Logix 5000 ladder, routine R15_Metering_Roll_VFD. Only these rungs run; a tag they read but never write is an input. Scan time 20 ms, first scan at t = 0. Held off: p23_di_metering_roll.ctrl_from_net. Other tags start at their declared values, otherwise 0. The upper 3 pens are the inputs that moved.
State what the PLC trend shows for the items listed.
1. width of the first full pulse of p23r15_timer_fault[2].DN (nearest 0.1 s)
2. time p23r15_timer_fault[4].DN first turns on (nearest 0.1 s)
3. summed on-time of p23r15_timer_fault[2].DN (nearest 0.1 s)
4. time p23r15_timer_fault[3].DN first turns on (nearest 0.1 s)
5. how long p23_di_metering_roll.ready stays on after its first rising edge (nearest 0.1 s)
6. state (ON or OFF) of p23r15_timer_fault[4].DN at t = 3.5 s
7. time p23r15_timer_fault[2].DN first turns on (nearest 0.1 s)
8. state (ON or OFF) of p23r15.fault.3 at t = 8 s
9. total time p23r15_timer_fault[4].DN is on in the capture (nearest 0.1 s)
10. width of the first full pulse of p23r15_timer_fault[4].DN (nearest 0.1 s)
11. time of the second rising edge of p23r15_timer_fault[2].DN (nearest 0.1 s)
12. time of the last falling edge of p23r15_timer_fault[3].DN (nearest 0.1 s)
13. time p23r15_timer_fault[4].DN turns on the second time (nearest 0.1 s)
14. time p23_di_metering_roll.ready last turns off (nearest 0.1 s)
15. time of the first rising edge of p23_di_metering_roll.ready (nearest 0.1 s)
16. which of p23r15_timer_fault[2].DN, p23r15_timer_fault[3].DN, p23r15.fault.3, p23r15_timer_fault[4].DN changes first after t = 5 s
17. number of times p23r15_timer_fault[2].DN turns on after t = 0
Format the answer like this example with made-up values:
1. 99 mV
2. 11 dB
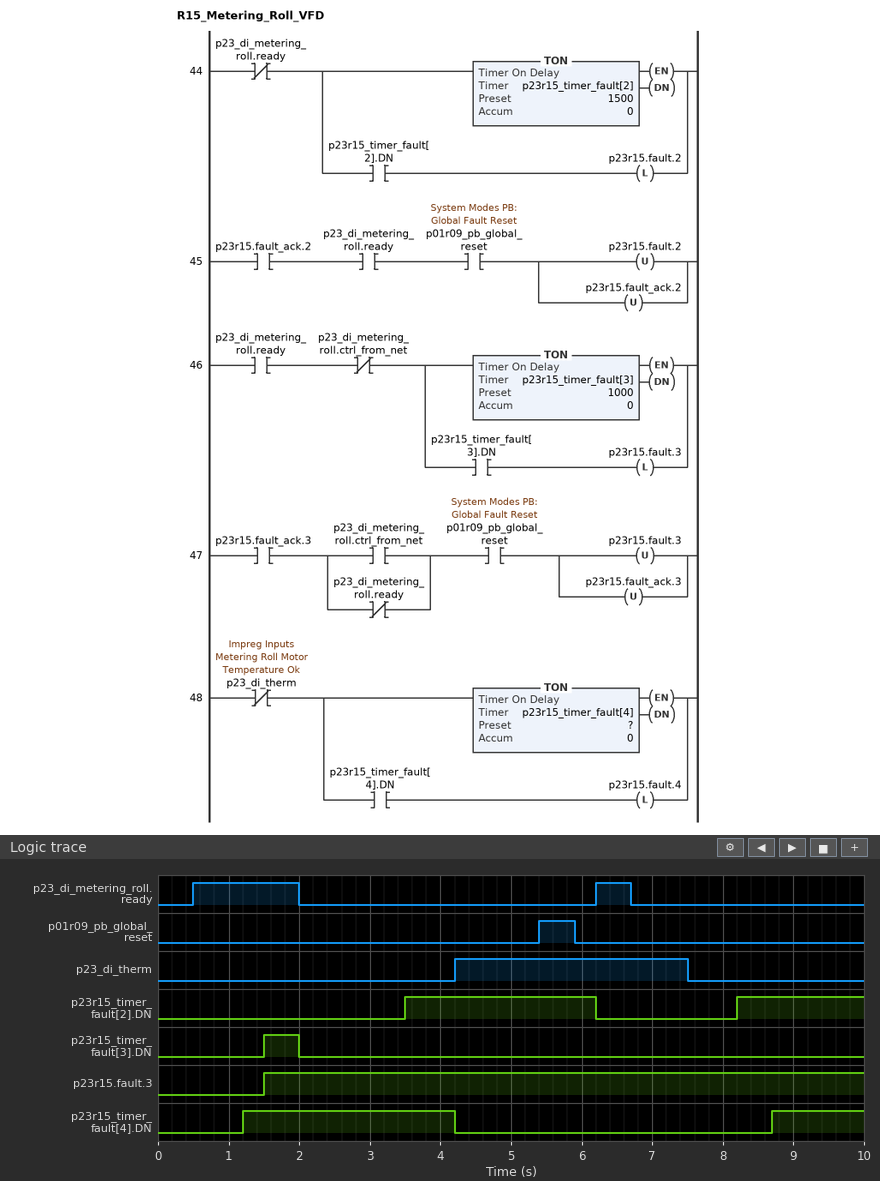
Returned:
1. 2.7 s
2. 1.2 s
3. 4.5 s
4. 1.5 s
5. 1.5 s
6. ON
7. 3.5 s
8. ON
9. 4.3 s
10. 3.0 s
11. 8.2 s
12. 2.0 s
13. 8.7 s
14. 6.7 s
15. 0.5 s
16. p23r15_timer_fault[2].DN
17. 2
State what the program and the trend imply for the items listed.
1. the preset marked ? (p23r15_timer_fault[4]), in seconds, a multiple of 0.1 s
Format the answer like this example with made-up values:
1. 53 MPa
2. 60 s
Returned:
1. 1.2 s
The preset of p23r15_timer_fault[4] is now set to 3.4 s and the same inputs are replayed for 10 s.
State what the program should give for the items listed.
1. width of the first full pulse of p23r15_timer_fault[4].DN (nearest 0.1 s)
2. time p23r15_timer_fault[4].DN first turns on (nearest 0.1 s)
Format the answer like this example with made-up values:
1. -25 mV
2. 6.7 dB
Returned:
1. 0.8 s
2. 3.4 s
